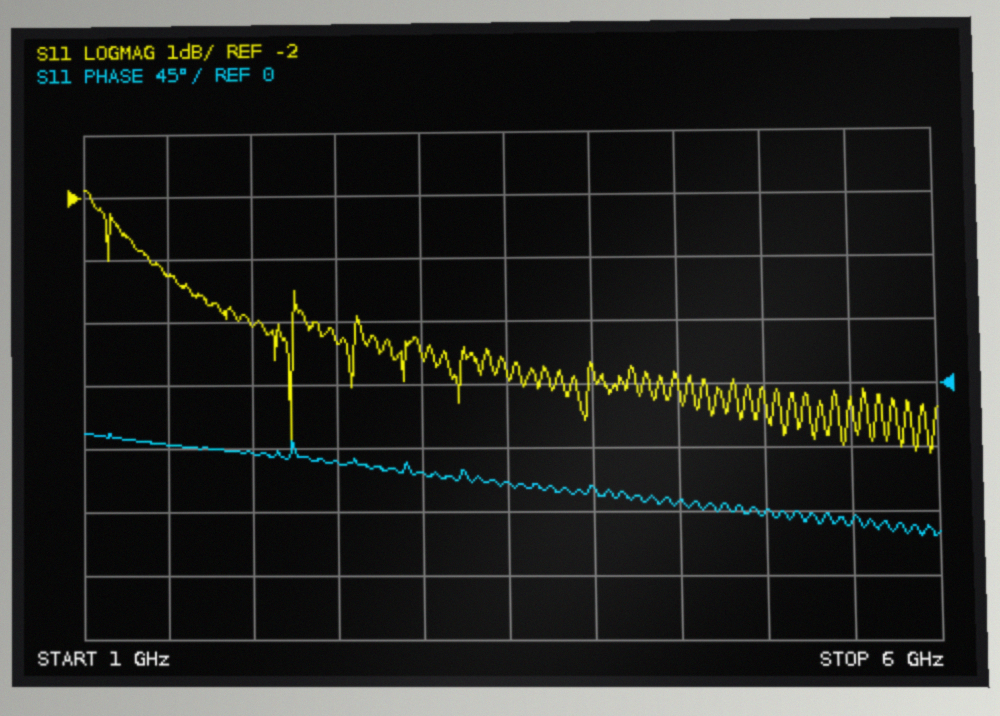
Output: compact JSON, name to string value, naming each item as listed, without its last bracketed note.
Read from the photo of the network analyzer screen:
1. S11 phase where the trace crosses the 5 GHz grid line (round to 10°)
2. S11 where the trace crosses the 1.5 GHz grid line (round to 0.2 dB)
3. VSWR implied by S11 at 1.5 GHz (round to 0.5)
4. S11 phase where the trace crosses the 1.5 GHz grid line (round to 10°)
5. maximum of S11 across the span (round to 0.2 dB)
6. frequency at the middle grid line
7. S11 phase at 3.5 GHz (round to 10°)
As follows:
{"S11 phase where the trace crosses the 5 GHz grid line": "-90°", "S11 where the trace crosses the 1.5 GHz grid line": "-3.2 dB", "VSWR implied by S11 at 1.5 GHz": "5.5", "S11 phase where the trace crosses the 1.5 GHz grid line": "-40°", "maximum of S11 across the span": "-1.8 dB", "frequency at the middle grid line": "3.5 GHz", "S11 phase at 3.5 GHz": "-70°"}
